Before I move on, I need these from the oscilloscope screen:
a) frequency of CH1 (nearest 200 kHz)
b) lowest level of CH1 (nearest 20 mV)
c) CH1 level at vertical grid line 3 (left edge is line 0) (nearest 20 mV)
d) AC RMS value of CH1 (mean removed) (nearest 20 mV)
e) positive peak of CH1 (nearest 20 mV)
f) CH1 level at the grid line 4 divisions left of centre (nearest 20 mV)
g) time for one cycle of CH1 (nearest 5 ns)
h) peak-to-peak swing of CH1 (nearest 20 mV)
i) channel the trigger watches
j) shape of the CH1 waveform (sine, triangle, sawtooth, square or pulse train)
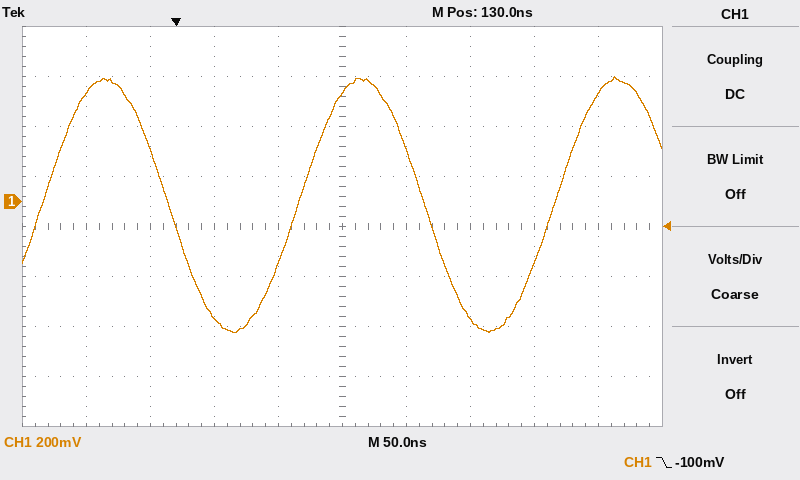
5.0 MHz
-520 mV
-460 mV
360 mV
500 mV
440 mV
200 ns
1.02 V
CH1
sine
